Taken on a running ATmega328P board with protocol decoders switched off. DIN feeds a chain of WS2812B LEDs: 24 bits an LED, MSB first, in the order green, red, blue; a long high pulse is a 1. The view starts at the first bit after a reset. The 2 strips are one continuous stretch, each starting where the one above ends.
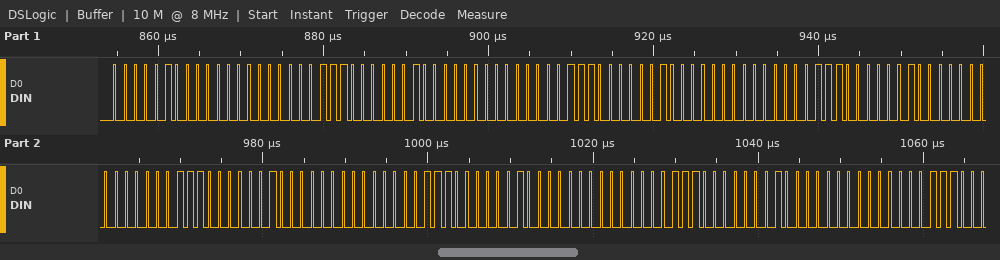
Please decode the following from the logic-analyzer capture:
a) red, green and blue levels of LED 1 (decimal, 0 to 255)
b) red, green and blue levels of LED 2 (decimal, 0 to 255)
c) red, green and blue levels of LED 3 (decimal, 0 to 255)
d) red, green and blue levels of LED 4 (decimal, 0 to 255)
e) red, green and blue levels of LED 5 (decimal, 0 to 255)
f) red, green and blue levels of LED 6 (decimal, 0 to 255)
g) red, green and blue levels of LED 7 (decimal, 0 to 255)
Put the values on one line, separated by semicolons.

0, 4, 14; 0, 4, 14; 0, 4, 14; 0, 4, 14; 0, 4, 14; 0, 4, 14; 0, 2, 7
